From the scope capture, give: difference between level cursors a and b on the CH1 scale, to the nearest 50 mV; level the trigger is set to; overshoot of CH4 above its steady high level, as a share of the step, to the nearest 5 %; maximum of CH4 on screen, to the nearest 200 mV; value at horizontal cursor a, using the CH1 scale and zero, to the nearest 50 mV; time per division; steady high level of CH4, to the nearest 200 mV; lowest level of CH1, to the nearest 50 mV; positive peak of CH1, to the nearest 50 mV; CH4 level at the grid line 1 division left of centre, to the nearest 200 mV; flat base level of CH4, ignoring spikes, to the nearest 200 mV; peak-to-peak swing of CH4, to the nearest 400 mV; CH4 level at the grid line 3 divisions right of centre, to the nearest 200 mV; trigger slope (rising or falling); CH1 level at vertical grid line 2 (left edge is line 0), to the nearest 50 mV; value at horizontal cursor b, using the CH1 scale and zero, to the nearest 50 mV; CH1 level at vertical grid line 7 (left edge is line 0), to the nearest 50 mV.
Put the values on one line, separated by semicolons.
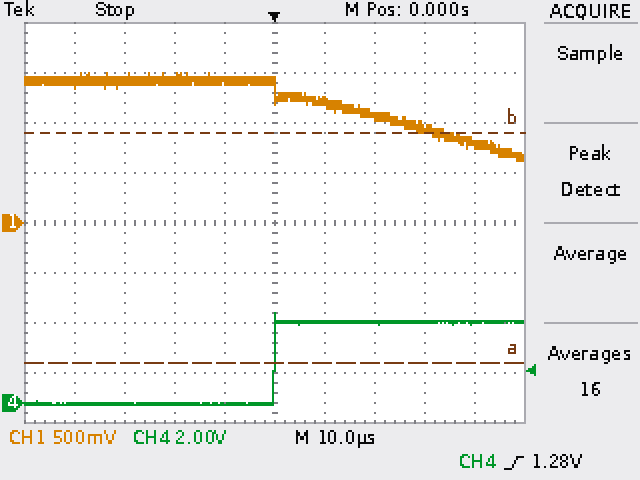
2.30 V; 1.28 V; 10 %; 3.6 V; -1.40 V; 10 µs; 3.2 V; 600 mV; 1.50 V; 0.0 V; 0.0 V; 3.6 V; 3.2 V; rising; 1.40 V; 900 mV; 1.05 V
